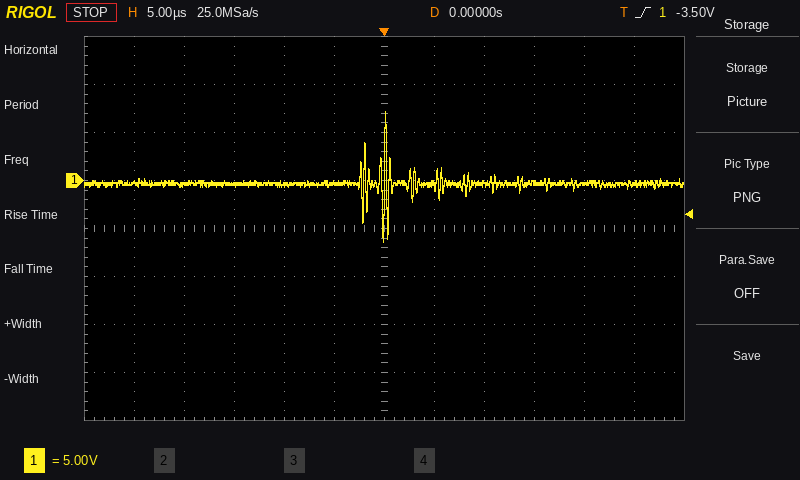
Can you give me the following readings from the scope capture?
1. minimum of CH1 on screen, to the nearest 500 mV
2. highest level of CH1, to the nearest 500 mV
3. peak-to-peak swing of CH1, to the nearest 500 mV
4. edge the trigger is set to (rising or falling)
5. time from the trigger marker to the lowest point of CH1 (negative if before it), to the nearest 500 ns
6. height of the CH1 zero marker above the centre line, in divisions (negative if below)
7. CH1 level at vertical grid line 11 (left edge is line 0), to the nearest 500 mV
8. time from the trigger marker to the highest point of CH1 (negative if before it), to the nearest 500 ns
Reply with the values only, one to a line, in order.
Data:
-6.5 V
7.0 V
13.5 V
rising
0.0 µs
+1.0 div
-500 mV
0.0 µs
